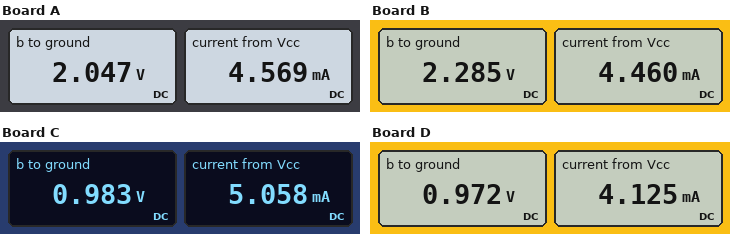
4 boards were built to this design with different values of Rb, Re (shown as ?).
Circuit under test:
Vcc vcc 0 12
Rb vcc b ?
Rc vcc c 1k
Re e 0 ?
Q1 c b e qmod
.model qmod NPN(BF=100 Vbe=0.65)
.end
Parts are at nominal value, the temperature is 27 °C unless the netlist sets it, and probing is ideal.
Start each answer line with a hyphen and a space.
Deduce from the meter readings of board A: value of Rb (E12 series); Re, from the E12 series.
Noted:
- 220 kΩ
- 270 Ω
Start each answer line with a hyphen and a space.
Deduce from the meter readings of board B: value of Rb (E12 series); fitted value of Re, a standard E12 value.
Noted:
- 220 kΩ
- 330 Ω
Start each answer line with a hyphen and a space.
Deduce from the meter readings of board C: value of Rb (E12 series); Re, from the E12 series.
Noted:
- 220 kΩ
- 33 Ω
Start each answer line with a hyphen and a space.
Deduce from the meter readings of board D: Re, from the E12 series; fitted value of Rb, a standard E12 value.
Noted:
- 39 Ω
- 270 kΩ
